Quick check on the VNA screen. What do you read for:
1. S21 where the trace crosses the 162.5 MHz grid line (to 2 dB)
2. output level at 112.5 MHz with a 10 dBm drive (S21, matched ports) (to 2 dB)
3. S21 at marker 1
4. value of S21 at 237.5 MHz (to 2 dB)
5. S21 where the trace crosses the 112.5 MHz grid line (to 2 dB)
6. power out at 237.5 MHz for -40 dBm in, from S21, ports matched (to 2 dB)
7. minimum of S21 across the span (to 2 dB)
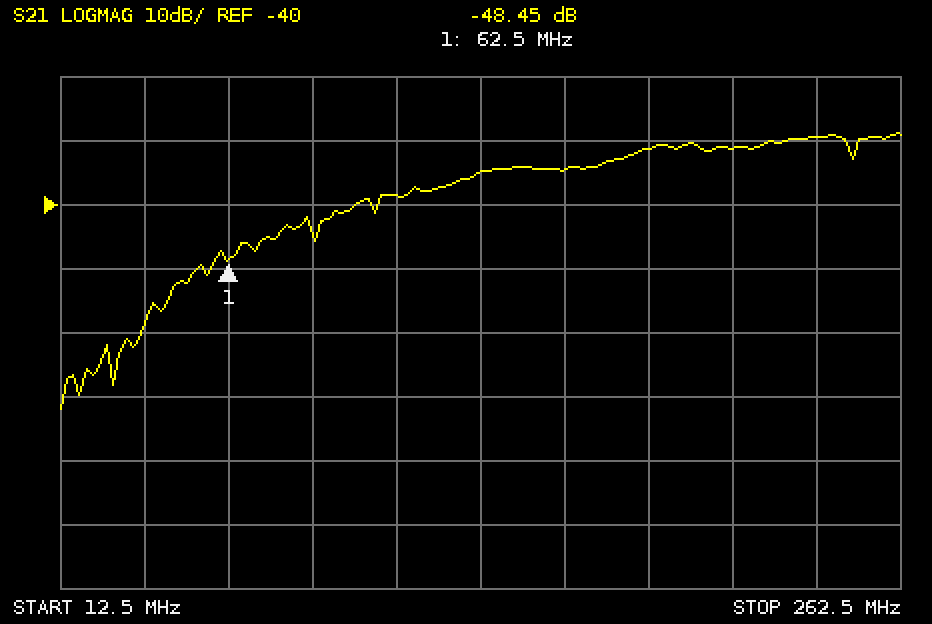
-34 dB
-28 dBm
-48.45 dB
-30 dB
-38 dB
-70 dBm
-72 dB
